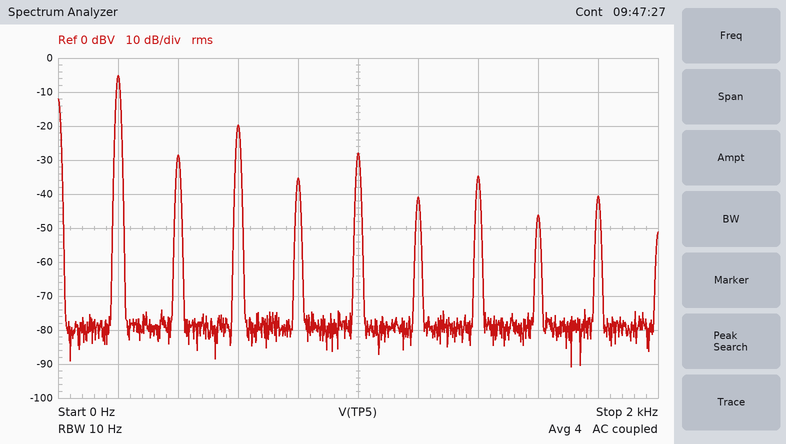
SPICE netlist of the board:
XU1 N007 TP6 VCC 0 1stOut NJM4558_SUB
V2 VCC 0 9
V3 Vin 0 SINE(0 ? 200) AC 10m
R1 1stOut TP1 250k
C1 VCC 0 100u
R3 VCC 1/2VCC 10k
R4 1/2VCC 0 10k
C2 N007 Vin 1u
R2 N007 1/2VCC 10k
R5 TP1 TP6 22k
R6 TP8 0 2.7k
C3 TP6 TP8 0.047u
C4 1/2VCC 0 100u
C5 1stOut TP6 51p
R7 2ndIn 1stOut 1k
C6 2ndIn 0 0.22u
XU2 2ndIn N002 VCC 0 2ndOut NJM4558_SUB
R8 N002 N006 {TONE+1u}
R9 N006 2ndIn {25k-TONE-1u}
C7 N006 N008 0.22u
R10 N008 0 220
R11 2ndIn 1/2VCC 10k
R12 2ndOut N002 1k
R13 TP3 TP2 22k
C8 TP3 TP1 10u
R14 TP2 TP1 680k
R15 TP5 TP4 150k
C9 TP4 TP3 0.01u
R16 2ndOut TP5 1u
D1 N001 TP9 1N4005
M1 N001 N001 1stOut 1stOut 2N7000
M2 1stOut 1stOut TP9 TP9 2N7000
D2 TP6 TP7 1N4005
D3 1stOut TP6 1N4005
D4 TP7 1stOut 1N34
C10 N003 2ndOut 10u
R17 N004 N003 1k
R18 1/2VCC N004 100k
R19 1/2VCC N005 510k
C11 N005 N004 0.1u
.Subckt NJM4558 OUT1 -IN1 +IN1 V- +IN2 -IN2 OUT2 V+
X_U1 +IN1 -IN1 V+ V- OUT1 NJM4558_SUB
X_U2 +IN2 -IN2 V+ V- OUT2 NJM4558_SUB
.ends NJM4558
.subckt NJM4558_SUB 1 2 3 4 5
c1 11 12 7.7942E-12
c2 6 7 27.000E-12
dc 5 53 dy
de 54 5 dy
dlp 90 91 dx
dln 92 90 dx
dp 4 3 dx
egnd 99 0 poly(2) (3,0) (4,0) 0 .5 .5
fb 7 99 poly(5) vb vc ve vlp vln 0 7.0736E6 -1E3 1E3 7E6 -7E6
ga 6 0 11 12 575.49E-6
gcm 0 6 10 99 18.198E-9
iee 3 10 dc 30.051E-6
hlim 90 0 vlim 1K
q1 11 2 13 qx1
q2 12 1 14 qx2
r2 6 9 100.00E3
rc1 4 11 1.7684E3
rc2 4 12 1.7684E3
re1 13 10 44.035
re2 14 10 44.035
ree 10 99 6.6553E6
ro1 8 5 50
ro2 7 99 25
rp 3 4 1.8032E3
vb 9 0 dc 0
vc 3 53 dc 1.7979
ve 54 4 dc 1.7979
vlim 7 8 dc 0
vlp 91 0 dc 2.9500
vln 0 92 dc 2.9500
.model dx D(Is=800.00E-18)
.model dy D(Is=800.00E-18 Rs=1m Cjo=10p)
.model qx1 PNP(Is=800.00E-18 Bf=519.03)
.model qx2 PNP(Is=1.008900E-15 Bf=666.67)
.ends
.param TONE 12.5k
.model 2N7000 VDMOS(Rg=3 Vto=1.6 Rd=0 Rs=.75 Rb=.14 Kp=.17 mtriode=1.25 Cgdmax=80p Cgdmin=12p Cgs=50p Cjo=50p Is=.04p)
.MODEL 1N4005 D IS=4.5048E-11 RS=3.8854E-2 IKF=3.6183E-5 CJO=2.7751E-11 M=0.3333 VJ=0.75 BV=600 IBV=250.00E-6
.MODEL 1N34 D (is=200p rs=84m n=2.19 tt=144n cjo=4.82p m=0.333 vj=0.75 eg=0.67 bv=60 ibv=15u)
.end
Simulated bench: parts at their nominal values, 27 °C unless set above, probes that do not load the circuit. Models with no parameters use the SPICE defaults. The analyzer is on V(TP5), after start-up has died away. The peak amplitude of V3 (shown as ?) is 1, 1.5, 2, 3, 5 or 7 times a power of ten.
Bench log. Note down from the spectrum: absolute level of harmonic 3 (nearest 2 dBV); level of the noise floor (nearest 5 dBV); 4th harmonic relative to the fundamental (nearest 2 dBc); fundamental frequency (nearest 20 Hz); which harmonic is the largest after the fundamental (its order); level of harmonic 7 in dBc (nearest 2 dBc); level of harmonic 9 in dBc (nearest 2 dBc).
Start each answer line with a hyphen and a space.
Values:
- -20 dBV
- -80 dBV
- -30 dBc
- 200 Hz
- 3
- -30 dBc
- -36 dBc
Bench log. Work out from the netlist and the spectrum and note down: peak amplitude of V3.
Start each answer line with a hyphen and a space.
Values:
- 300 mV
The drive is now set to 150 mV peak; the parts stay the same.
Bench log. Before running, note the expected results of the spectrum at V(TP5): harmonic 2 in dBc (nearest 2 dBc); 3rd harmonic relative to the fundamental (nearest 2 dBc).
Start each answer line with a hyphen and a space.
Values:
- -20 dBc
- -16 dBc
